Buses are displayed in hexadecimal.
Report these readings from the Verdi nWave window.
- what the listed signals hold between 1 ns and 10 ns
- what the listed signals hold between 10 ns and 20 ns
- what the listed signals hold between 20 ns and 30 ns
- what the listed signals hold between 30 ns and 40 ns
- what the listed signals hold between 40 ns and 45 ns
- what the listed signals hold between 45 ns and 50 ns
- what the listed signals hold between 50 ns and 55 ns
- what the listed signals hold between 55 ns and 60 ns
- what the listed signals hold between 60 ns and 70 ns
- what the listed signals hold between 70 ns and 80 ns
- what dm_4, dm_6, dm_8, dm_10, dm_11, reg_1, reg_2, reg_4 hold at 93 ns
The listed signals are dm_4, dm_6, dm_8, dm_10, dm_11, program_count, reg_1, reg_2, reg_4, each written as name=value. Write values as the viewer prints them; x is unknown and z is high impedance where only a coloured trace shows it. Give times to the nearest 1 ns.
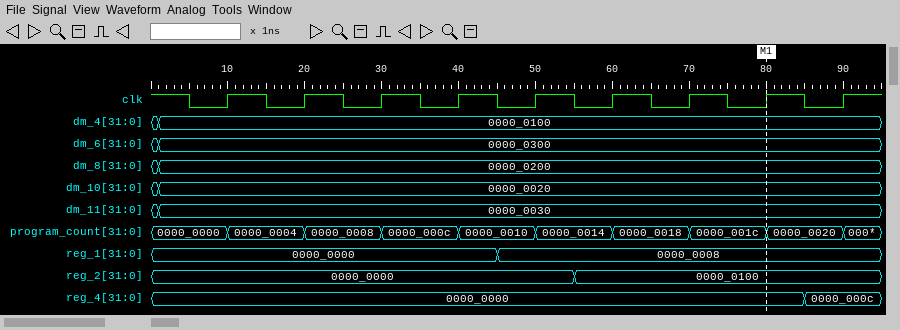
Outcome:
dm_4=0000_0100, dm_6=0000_0300, dm_8=0000_0200, dm_10=0000_0020, dm_11=0000_0030, program_count=0000_0000, reg_1=0000_0000, reg_2=0000_0000, reg_4=0000_0000
dm_4=0000_0100, dm_6=0000_0300, dm_8=0000_0200, dm_10=0000_0020, dm_11=0000_0030, program_count=0000_0004, reg_1=0000_0000, reg_2=0000_0000, reg_4=0000_0000
dm_4=0000_0100, dm_6=0000_0300, dm_8=0000_0200, dm_10=0000_0020, dm_11=0000_0030, program_count=0000_0008, reg_1=0000_0000, reg_2=0000_0000, reg_4=0000_0000
dm_4=0000_0100, dm_6=0000_0300, dm_8=0000_0200, dm_10=0000_0020, dm_11=0000_0030, program_count=0000_000c, reg_1=0000_0000, reg_2=0000_0000, reg_4=0000_0000
dm_4=0000_0100, dm_6=0000_0300, dm_8=0000_0200, dm_10=0000_0020, dm_11=0000_0030, program_count=0000_0010, reg_1=0000_0000, reg_2=0000_0000, reg_4=0000_0000
dm_4=0000_0100, dm_6=0000_0300, dm_8=0000_0200, dm_10=0000_0020, dm_11=0000_0030, program_count=0000_0010, reg_1=0000_0008, reg_2=0000_0000, reg_4=0000_0000
dm_4=0000_0100, dm_6=0000_0300, dm_8=0000_0200, dm_10=0000_0020, dm_11=0000_0030, program_count=0000_0014, reg_1=0000_0008, reg_2=0000_0000, reg_4=0000_0000
dm_4=0000_0100, dm_6=0000_0300, dm_8=0000_0200, dm_10=0000_0020, dm_11=0000_0030, program_count=0000_0014, reg_1=0000_0008, reg_2=0000_0100, reg_4=0000_0000
dm_4=0000_0100, dm_6=0000_0300, dm_8=0000_0200, dm_10=0000_0020, dm_11=0000_0030, program_count=0000_0018, reg_1=0000_0008, reg_2=0000_0100, reg_4=0000_0000
dm_4=0000_0100, dm_6=0000_0300, dm_8=0000_0200, dm_10=0000_0020, dm_11=0000_0030, program_count=0000_001c, reg_1=0000_0008, reg_2=0000_0100, reg_4=0000_0000
dm_4=0000_0100, dm_6=0000_0300, dm_8=0000_0200, dm_10=0000_0020, dm_11=0000_0030, reg_1=0000_0008, reg_2=0000_0100, reg_4=0000_000c
